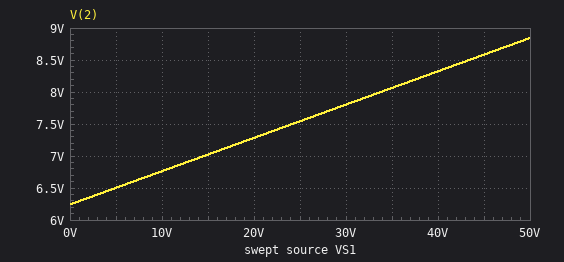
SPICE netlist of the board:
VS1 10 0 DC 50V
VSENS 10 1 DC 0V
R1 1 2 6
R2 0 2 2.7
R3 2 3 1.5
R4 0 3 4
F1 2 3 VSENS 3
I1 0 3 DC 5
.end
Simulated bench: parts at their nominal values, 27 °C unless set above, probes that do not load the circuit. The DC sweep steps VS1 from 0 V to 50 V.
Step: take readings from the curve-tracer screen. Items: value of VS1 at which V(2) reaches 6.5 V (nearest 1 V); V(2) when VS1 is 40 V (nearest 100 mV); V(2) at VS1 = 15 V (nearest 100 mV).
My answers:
5 V
8.3 V
7.0 V
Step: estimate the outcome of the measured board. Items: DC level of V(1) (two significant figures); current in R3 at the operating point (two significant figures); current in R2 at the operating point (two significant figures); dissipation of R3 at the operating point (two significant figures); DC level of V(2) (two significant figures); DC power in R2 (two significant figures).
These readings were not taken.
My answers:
50 V
17 A
3.3 A
430 W
8.8 V
29 W
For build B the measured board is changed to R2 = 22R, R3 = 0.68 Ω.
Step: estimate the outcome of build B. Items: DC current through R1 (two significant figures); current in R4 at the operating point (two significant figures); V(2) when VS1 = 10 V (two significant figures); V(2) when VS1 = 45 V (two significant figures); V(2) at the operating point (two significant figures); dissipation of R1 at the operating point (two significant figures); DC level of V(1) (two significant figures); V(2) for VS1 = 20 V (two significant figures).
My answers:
4.1 A
7.9 A
15 V
24 V
25 V
100 W
50 V
17 V
